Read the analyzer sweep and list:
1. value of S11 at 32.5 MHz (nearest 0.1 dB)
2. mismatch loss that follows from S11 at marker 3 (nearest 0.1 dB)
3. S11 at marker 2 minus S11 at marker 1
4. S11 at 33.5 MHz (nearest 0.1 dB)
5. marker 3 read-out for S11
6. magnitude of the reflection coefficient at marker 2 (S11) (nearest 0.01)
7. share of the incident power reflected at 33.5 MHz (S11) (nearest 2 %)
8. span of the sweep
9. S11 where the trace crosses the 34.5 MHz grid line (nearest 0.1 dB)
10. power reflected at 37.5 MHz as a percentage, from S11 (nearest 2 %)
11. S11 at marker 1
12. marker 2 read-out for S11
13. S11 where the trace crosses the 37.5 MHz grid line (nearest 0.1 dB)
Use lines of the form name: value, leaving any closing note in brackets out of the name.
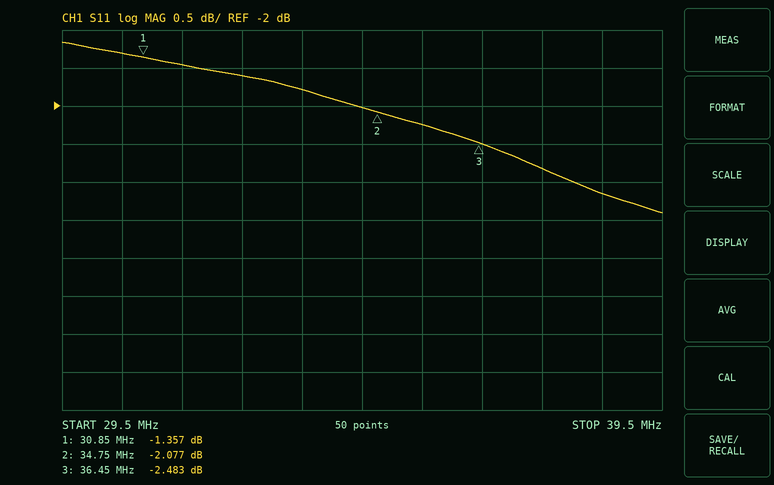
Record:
value of S11 at 32.5 MHz: -1.6 dB
mismatch loss that follows from S11 at marker 3: 3.6 dB
S11 at marker 2 minus S11 at marker 1: -0.720 dB
S11 at 33.5 MHz: -1.8 dB
marker 3 read-out for S11: -2.483 dB
magnitude of the reflection coefficient at marker 2 (S11): 0.79
share of the incident power reflected at 33.5 MHz (S11): 66 %
span of the sweep: 10 MHz
S11 where the trace crosses the 34.5 MHz grid line: -2.0 dB
power reflected at 37.5 MHz as a percentage, from S11: 52 %
S11 at marker 1: -1.357 dB
marker 2 read-out for S11: -2.077 dB
S11 where the trace crosses the 37.5 MHz grid line: -2.8 dB
